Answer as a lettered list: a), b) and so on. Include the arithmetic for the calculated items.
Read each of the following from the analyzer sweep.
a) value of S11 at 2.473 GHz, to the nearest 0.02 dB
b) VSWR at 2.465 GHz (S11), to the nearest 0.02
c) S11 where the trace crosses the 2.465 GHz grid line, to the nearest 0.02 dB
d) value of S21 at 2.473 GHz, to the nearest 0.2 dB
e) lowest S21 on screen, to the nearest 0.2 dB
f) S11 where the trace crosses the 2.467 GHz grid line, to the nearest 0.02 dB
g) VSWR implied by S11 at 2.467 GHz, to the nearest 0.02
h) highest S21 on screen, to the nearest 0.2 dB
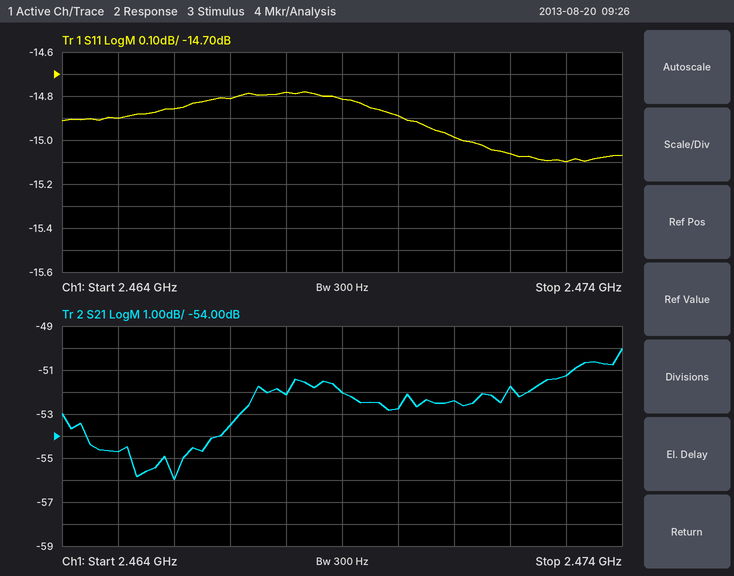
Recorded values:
a) -15.10 dB
b) |Γ| = 10^(-14.9/20) = 0.1799; VSWR = (1 + 0.1799)/(1 − 0.1799) ≈ 1.44
c) -14.90 dB
d) -51.2 dB
e) -56.0 dB
f) -14.82 dB
g) |Γ| = 10^(-14.82/20) = 0.1816; VSWR = (1 + 0.1816)/(1 − 0.1816) ≈ 1.44
h) -50.0 dB
